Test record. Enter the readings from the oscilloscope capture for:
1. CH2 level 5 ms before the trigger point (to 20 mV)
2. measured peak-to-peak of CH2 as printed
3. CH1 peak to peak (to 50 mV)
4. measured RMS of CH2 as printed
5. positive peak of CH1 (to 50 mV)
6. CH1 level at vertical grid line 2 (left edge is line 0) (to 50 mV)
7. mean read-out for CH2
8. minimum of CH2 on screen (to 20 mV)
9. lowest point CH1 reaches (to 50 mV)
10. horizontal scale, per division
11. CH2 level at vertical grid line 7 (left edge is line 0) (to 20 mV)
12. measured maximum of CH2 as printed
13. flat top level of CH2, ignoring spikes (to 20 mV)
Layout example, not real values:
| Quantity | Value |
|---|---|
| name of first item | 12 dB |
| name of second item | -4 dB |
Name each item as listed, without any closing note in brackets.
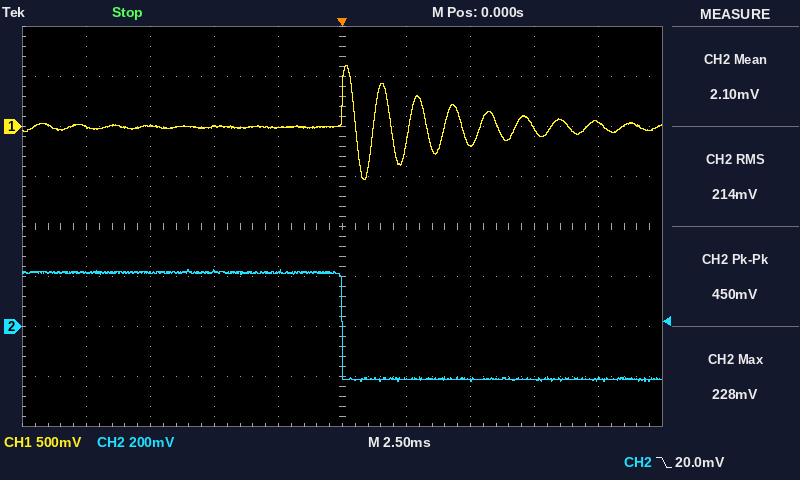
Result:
| Quantity | Value |
|---|---|
| CH2 level 5 ms before the trigger point | 220 mV |
| measured peak-to-peak of CH2 as printed | 450 mV |
| CH1 peak to peak | 1.15 V |
| measured RMS of CH2 as printed | 214 mV |
| positive peak of CH1 | 600 mV |
| CH1 level at vertical grid line 2 (left edge is line 0) | 0 mV |
| mean read-out for CH2 | 2.10 mV |
| minimum of CH2 on screen | -220 mV |
| lowest point CH1 reaches | -550 mV |
| horizontal scale, per division | 2.5 ms |
| CH2 level at vertical grid line 7 (left edge is line 0) | -220 mV |
| measured maximum of CH2 as printed | 228 mV |
| flat top level of CH2, ignoring spikes | 220 mV |
